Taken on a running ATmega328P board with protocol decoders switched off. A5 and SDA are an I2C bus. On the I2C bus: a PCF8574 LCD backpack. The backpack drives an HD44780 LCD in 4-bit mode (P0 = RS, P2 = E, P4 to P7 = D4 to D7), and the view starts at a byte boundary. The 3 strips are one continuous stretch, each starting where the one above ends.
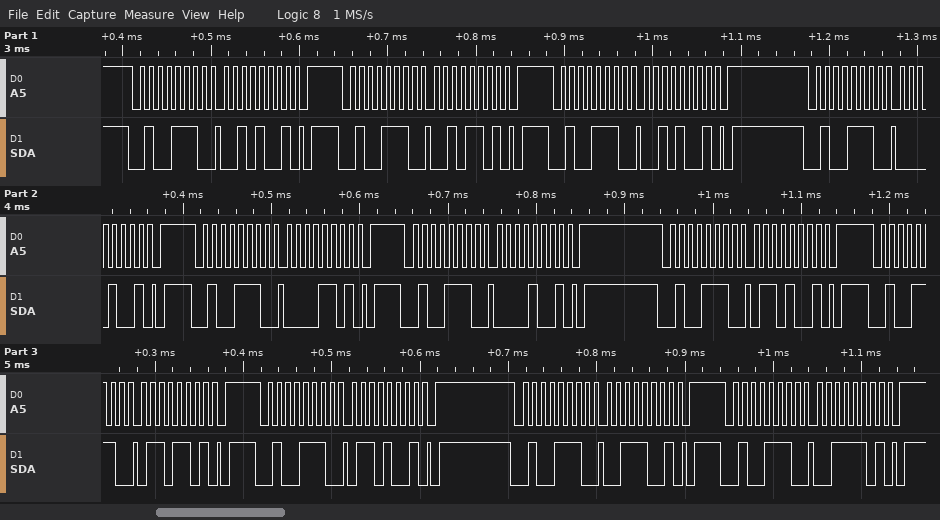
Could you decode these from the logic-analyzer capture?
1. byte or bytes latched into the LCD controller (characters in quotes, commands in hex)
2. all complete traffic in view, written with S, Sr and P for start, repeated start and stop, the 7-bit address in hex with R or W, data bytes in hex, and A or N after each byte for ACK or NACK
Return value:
' '
S 27W A 29 A P S 27W A 2D A P S 27W A 29 A P S 27W A 09 A P S 27W A 0D A P S 27W A 09 A P S 27W A 69 A P S 27W A 6D A P S 27W A 69 A P S 27W A 39 A P S 27W A 3D A P
